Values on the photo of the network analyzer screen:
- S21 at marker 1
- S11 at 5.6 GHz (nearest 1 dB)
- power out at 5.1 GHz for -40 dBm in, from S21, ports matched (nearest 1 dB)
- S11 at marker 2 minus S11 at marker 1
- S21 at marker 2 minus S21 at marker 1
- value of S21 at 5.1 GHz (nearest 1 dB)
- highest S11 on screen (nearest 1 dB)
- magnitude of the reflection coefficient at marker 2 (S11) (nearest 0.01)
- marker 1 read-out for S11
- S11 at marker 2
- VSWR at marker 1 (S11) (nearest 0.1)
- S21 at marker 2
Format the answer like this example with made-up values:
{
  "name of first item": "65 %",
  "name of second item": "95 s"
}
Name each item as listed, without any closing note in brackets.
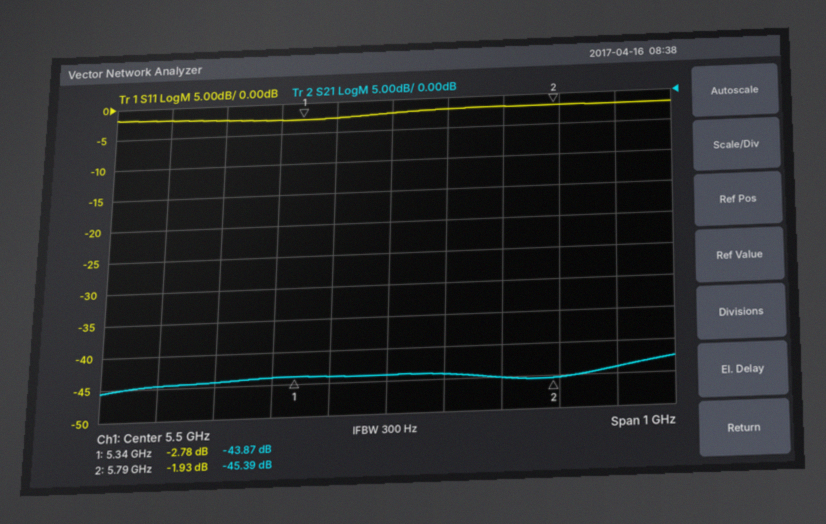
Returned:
{
  "S21 at marker 1": "-43.87 dB",
  "S11 at 5.6 GHz": "-2 dB",
  "power out at 5.1 GHz for -40 dBm in, from S21, ports matched": "-85 dBm",
  "S11 at marker 2 minus S11 at marker 1": "0.85 dB",
  "S21 at marker 2 minus S21 at marker 1": "-1.52 dB",
  "value of S21 at 5.1 GHz": "-45 dB",
  "highest S11 on screen": "-2 dB",
  "magnitude of the reflection coefficient at marker 2 (S11)": "0.80",
  "marker 1 read-out for S11": "-2.78 dB",
  "S11 at marker 2": "-1.93 dB",
  "VSWR at marker 1 (S11)": "6.3",
  "S21 at marker 2": "-45.39 dB"
}
